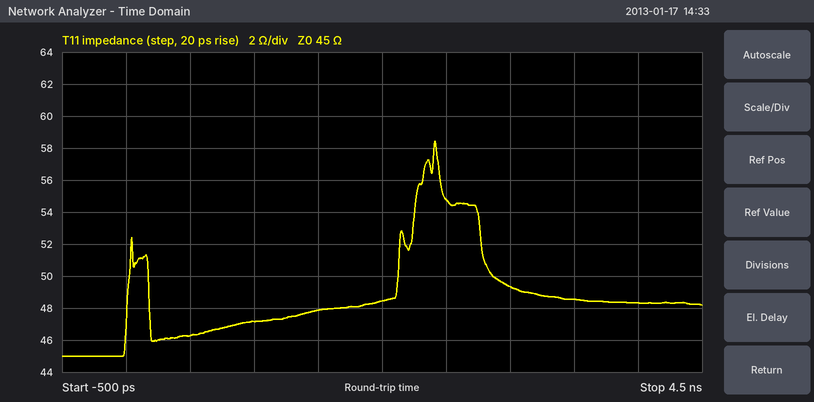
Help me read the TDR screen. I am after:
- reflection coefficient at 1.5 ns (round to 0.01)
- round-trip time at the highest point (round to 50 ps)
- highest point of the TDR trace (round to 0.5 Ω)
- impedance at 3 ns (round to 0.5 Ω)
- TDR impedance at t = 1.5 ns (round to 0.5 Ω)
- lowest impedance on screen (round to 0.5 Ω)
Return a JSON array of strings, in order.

["+0.03", "2.40 ns", "58.5 Ω", "49.5 Ω", "48.0 Ω", "45.0 Ω"]
